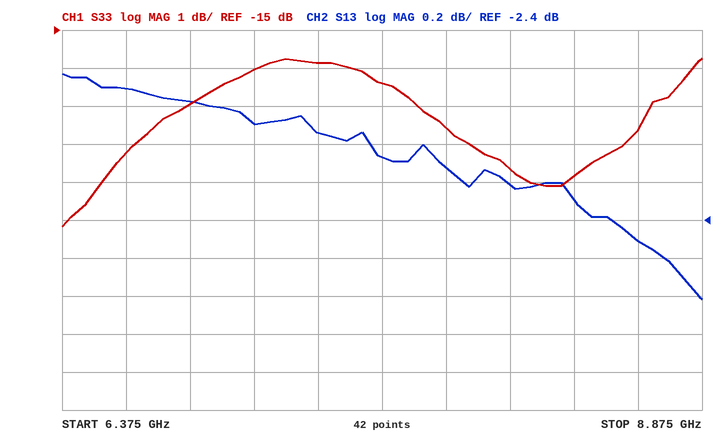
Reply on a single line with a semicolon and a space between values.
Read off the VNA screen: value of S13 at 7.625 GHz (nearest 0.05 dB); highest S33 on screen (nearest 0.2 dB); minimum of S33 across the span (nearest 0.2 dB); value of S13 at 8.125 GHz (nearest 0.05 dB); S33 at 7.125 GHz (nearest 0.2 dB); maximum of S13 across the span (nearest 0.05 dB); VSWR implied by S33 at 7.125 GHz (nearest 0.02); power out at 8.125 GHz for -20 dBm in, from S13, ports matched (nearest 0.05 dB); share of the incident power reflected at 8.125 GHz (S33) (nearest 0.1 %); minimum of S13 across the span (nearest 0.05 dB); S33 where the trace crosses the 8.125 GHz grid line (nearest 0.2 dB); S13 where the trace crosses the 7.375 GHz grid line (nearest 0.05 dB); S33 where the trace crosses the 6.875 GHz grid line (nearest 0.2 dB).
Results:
-2.05 dB; -15.8 dB; -20.2 dB; -2.20 dB; -16.0 dB; -1.65 dB; 1.38; -22.20 dBm; 1.4 %; -2.80 dB; -18.6 dB; -1.95 dB; -17.0 dB
